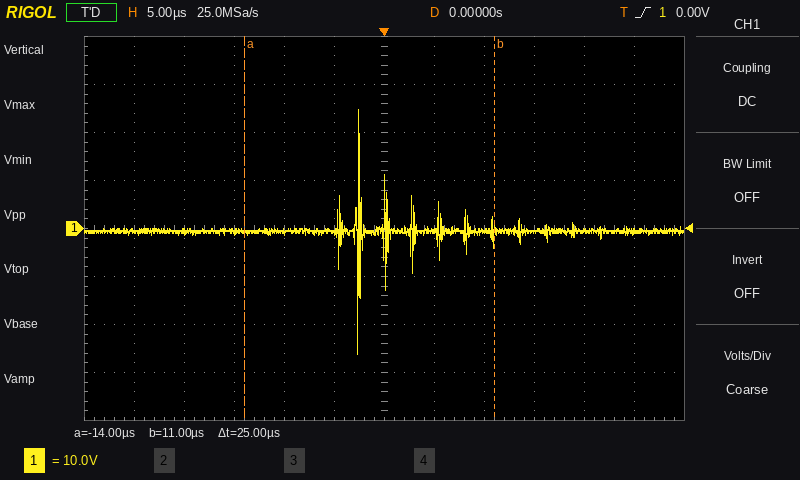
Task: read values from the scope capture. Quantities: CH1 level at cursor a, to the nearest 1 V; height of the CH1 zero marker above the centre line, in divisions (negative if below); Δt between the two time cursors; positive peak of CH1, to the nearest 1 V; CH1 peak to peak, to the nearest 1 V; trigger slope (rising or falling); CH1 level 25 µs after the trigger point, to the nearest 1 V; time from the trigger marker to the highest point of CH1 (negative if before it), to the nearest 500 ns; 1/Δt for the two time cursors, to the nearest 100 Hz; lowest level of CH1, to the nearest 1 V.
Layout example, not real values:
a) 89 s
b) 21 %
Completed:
a) -1 V
b) 0.0 div
c) 25 µs
d) 25 V
e) 51 V
f) rising
g) -1 V
h) -2.5 µs
i) 40.0 kHz
j) -26 V
